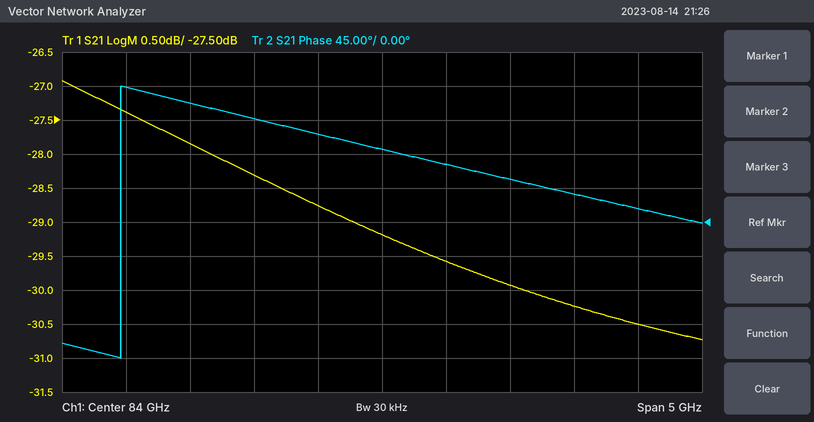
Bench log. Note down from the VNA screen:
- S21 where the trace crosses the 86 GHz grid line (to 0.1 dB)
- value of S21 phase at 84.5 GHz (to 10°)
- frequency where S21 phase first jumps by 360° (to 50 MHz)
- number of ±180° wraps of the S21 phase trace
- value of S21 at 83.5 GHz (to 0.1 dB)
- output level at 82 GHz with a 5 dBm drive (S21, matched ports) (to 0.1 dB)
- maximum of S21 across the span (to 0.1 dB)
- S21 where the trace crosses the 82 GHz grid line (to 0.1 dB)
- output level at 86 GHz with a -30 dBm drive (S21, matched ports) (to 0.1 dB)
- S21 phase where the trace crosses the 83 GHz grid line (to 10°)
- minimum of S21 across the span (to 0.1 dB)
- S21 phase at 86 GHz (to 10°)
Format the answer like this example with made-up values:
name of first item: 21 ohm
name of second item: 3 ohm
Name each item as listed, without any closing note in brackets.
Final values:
S21 where the trace crosses the 86 GHz grid line: -30.5 dB
value of S21 phase at 84.5 GHz: 80°
frequency where S21 phase first jumps by 360°: 81.95 GHz
number of ±180° wraps of the S21 phase trace: 1
value of S21 at 83.5 GHz: -28.8 dB
output level at 82 GHz with a 5 dBm drive (S21, matched ports): -22.4 dBm
maximum of S21 across the span: -26.9 dB
S21 where the trace crosses the 82 GHz grid line: -27.4 dB
output level at 86 GHz with a -30 dBm drive (S21, matched ports): -60.5 dBm
S21 phase where the trace crosses the 83 GHz grid line: 140°
minimum of S21 across the span: -30.7 dB
S21 phase at 86 GHz: 20°
